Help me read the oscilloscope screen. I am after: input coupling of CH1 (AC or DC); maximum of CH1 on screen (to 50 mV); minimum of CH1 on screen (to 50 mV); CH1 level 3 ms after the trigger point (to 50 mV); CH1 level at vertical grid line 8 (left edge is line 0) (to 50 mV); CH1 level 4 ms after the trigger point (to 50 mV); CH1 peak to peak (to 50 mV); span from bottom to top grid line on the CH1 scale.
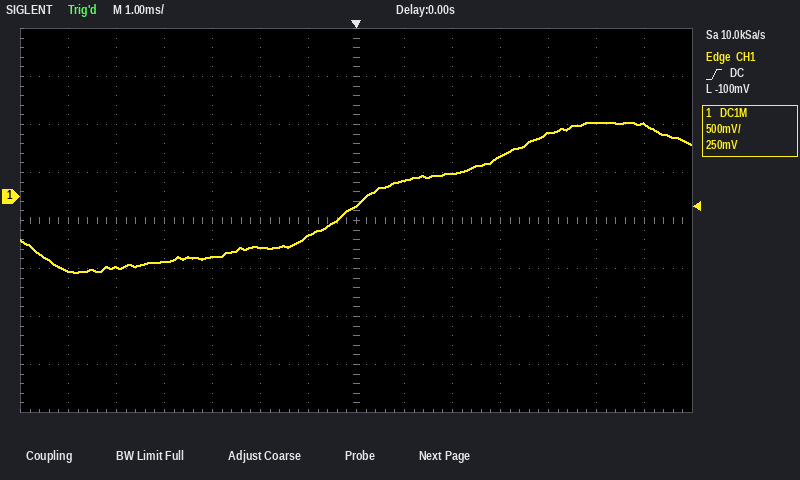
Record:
DC
750 mV
-800 mV
400 mV
150 mV
650 mV
1.55 V
4 V
